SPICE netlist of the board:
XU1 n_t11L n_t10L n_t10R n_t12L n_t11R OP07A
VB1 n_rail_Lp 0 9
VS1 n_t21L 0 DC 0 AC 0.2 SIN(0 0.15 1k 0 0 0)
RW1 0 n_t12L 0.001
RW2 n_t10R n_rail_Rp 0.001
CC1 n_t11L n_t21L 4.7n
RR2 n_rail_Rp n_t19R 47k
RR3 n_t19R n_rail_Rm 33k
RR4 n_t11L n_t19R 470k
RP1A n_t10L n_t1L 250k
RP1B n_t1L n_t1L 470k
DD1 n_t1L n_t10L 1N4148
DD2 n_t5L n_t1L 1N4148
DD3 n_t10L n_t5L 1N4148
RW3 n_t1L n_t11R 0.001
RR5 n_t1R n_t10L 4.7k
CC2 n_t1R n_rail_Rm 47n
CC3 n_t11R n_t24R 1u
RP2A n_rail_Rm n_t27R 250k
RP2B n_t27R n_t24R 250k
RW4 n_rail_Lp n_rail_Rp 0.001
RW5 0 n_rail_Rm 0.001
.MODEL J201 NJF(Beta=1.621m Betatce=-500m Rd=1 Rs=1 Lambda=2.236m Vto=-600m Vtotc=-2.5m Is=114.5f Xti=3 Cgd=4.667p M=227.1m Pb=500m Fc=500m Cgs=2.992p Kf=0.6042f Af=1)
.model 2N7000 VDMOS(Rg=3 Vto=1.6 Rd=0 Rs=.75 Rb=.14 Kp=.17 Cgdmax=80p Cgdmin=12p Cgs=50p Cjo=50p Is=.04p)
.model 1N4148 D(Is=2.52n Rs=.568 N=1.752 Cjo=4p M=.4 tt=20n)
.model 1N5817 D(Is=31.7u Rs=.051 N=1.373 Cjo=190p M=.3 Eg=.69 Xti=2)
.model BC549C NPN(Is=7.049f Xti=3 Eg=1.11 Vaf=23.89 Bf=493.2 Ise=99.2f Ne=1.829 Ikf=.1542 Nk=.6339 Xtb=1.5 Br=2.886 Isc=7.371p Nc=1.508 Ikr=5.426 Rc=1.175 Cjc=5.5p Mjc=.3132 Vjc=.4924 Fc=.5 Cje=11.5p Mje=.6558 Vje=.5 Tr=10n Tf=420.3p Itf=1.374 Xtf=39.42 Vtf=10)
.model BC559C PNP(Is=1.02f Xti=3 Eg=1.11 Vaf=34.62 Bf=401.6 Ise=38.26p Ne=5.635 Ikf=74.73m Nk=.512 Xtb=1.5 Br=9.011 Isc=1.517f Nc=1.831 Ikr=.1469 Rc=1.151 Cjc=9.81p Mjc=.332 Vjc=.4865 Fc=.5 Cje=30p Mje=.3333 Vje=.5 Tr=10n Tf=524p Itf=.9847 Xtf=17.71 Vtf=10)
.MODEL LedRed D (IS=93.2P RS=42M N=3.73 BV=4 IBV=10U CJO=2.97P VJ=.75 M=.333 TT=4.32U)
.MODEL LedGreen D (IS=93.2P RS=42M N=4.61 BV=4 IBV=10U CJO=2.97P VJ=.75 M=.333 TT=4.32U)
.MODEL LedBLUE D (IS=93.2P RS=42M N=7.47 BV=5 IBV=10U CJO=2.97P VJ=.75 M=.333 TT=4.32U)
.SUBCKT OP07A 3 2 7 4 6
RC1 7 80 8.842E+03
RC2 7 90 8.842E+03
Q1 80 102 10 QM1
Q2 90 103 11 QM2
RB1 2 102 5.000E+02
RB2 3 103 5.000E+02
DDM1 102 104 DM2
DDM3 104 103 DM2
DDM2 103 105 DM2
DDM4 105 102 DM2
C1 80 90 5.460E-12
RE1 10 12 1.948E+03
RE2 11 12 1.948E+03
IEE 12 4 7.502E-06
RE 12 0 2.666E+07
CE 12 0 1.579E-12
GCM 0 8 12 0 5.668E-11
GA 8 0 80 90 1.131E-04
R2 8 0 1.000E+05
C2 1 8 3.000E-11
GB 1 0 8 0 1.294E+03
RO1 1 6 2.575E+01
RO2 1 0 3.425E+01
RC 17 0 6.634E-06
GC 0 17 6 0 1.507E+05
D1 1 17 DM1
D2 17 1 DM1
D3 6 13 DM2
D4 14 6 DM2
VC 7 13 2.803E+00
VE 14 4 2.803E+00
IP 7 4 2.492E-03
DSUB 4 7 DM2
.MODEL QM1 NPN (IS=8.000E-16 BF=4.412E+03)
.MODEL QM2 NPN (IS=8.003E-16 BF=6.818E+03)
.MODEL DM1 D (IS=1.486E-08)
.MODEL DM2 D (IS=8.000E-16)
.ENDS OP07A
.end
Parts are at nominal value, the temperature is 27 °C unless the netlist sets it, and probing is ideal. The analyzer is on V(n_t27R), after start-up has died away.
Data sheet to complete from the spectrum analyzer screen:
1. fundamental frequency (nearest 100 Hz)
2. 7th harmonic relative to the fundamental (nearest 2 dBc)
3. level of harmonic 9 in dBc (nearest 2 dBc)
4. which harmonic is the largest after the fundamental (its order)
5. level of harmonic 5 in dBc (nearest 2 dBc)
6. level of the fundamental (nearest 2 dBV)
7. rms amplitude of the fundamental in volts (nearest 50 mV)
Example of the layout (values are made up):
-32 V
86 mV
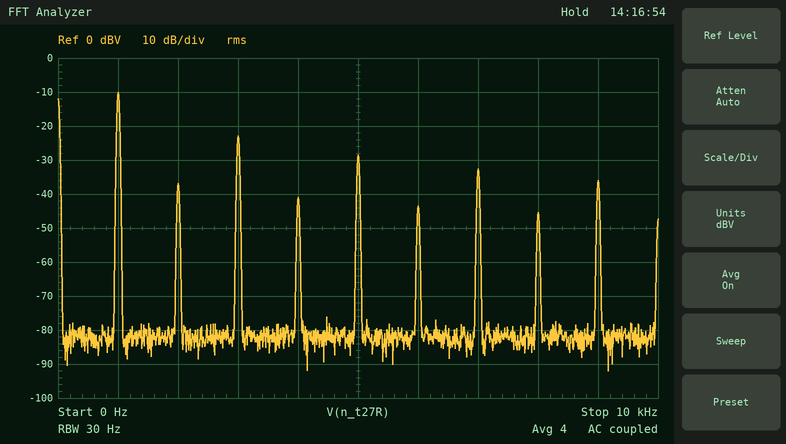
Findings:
1.0 kHz
-22 dBc
-26 dBc
3
-18 dBc
-10 dBV
300 mV
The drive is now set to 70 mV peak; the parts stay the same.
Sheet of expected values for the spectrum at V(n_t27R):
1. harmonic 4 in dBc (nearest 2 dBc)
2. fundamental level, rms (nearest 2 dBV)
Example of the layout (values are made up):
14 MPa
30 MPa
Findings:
-28 dBc
-12 dBV
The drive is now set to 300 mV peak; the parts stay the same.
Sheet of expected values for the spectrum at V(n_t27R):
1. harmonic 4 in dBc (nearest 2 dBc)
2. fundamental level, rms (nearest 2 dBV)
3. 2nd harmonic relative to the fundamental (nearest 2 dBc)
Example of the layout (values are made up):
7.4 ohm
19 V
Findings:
-34 dBc
-8 dBV
-30 dBc
